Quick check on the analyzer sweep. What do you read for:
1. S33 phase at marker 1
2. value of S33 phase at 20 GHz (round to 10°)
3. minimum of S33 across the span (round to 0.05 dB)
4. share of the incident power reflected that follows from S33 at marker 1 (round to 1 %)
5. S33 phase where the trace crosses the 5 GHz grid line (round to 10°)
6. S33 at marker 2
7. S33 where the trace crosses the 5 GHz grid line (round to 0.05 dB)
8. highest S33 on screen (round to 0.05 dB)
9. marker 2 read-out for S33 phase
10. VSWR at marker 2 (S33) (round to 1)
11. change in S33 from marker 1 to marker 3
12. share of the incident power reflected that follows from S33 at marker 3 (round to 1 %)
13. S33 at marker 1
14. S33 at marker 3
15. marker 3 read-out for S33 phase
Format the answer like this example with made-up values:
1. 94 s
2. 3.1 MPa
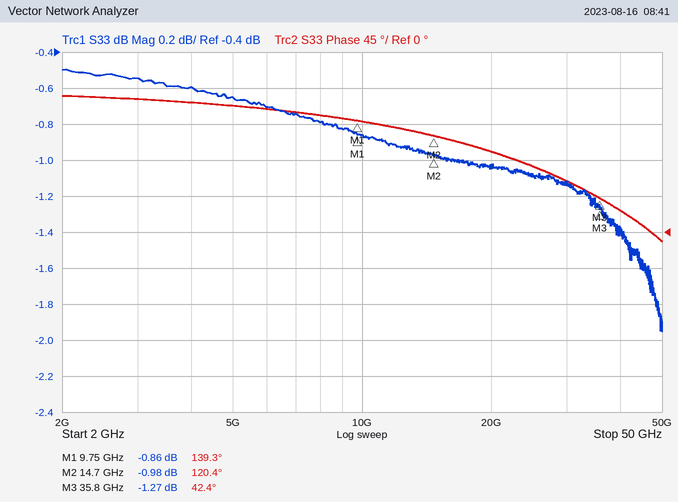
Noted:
1. 139.3°
2. 100°
3. -1.95 dB
4. 82 %
5. 160°
6. -0.98 dB
7. -0.65 dB
8. -0.50 dB
9. 120.4°
10. 18
11. -0.41 dB
12. 75 %
13. -0.86 dB
14. -1.27 dB
15. 42.4°
